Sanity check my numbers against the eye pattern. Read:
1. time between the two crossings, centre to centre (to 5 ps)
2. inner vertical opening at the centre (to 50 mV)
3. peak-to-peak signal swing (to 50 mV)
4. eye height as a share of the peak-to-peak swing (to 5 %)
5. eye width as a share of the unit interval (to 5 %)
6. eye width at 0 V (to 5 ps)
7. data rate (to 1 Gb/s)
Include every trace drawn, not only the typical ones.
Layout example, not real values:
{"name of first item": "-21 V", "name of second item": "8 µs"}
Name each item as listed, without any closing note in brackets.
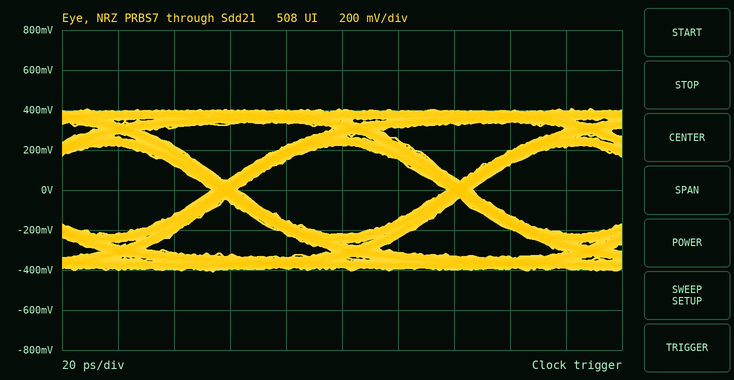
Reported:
{"time between the two crossings, centre to centre": "85 ps", "inner vertical opening at the centre": "450 mV", "peak-to-peak signal swing": "800 mV", "eye height as a share of the peak-to-peak swing": "55 %", "eye width as a share of the unit interval": "90 %", "eye width at 0 V": "75 ps", "data rate": "12 Gb/s"}
